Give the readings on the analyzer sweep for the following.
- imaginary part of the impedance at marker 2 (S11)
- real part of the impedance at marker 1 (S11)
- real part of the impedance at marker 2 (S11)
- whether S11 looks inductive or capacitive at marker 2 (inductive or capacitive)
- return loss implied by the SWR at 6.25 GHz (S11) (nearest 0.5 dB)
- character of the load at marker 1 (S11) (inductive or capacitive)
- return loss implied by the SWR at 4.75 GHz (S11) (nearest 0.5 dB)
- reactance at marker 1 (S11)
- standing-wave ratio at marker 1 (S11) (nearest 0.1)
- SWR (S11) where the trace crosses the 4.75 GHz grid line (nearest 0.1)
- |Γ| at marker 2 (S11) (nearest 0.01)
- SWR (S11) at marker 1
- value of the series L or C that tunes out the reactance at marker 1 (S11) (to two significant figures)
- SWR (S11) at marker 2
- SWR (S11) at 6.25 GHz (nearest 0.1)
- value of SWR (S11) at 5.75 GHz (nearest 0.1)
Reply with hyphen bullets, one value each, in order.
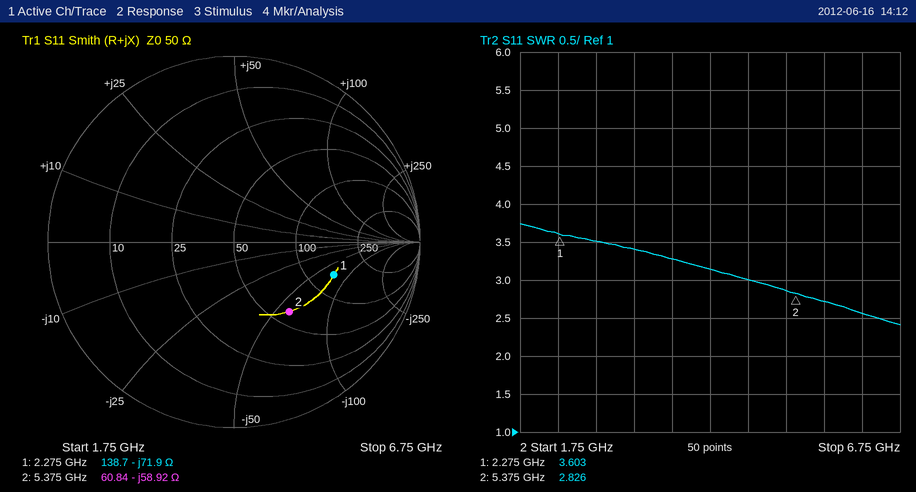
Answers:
- -58.92 Ω
- 138.7 Ω
- 60.84 Ω
- capacitive
- 7.0 dB
- capacitive
- 6.0 dB
- -71.9 Ω
- 3.6
- 3.0
- 0.48
- 3.603
- 5.0 nH
- 2.826
- 2.6
- 2.7
